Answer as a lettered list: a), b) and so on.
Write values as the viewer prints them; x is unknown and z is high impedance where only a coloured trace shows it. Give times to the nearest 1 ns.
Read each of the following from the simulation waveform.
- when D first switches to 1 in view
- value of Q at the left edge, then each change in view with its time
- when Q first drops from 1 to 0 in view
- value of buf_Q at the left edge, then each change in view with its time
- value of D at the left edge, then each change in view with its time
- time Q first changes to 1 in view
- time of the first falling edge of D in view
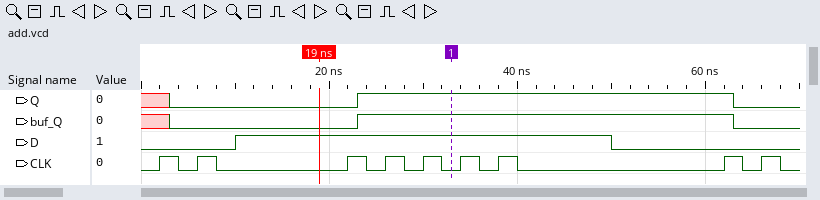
a) 10 ns
b) x, 0 at 3 ns, 1 at 23 ns, 0 at 63 ns
c) 63 ns
d) x, 0 at 3 ns, 1 at 23 ns, 0 at 63 ns
e) 0, 1 at 10 ns, 0 at 50 ns
f) 23 ns
g) 50 ns
